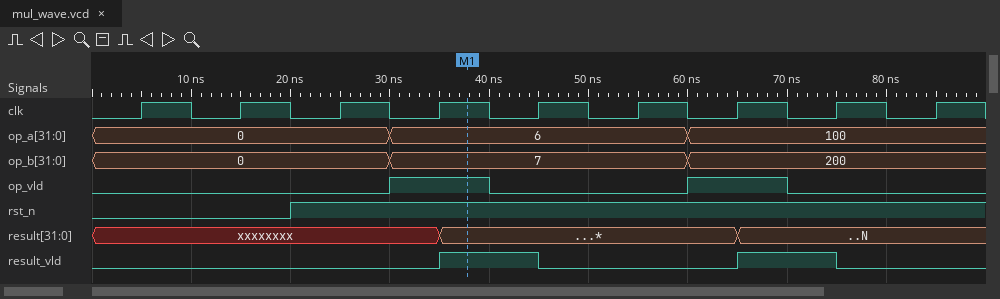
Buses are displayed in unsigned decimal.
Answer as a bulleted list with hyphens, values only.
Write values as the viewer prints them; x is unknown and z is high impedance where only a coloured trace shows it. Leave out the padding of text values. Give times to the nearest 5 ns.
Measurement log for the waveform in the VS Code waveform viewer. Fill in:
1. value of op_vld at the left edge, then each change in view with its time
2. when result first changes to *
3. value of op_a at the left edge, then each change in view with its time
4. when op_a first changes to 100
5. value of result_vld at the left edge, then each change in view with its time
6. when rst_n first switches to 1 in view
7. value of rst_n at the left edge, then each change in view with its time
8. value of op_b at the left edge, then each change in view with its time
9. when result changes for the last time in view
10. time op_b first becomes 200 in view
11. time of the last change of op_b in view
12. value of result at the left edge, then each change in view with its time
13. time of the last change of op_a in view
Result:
- 0, 1 at 30 ns, 0 at 40 ns, 1 at 60 ns, 0 at 70 ns
- 35 ns
- 0, 6 at 30 ns, 100 at 60 ns
- 60 ns
- 0, 1 at 35 ns, 0 at 45 ns, 1 at 65 ns, 0 at 75 ns
- 20 ns
- 0, 1 at 20 ns
- 0, 7 at 30 ns, 200 at 60 ns
- 65 ns
- 60 ns
- 60 ns
- xxxxxxxx, * at 35 ns, N at 65 ns
- 60 ns
